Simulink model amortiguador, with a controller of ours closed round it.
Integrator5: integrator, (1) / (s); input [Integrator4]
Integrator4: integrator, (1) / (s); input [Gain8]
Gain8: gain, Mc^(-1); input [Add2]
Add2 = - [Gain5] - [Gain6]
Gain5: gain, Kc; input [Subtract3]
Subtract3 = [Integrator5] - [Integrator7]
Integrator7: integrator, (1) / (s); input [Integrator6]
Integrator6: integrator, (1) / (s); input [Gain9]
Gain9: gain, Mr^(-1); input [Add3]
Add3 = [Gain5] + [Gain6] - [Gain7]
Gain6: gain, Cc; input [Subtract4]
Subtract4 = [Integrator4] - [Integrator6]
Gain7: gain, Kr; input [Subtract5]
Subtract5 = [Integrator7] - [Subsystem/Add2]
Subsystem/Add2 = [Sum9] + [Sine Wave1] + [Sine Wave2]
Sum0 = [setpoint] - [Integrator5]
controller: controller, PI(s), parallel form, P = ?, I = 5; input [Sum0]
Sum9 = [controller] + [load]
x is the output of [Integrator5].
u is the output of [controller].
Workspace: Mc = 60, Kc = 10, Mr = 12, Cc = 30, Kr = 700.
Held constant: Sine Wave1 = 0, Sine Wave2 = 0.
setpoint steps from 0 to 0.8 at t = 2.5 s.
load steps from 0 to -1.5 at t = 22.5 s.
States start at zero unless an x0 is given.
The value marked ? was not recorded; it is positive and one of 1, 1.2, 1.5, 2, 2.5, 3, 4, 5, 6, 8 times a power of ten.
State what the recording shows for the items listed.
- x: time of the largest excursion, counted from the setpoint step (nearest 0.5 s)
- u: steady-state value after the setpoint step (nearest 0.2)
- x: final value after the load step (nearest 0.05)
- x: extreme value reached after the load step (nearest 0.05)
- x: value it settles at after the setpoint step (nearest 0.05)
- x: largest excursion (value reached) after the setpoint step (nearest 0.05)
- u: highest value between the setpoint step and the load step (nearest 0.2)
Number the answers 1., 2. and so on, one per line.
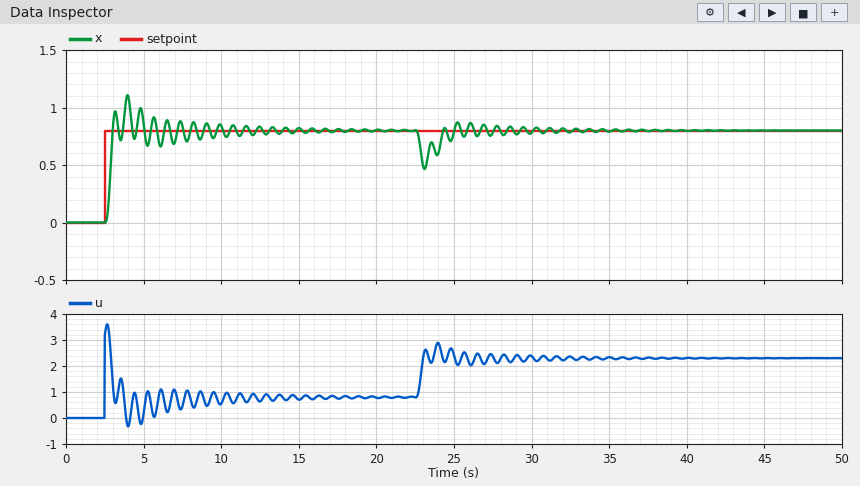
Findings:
1. 1.5 s
2. 0.8
3. 0.80
4. 0.45
5. 0.80
6. 1.10
7. 3.6
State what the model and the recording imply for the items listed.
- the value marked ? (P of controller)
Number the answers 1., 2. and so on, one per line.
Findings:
1. 4
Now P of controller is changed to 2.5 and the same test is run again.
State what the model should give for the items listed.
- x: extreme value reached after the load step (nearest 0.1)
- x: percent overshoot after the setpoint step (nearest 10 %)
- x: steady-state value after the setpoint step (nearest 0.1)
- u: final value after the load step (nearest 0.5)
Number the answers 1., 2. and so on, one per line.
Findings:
1. 0.4
2. 40 %
3. 0.8
4. 2.5
